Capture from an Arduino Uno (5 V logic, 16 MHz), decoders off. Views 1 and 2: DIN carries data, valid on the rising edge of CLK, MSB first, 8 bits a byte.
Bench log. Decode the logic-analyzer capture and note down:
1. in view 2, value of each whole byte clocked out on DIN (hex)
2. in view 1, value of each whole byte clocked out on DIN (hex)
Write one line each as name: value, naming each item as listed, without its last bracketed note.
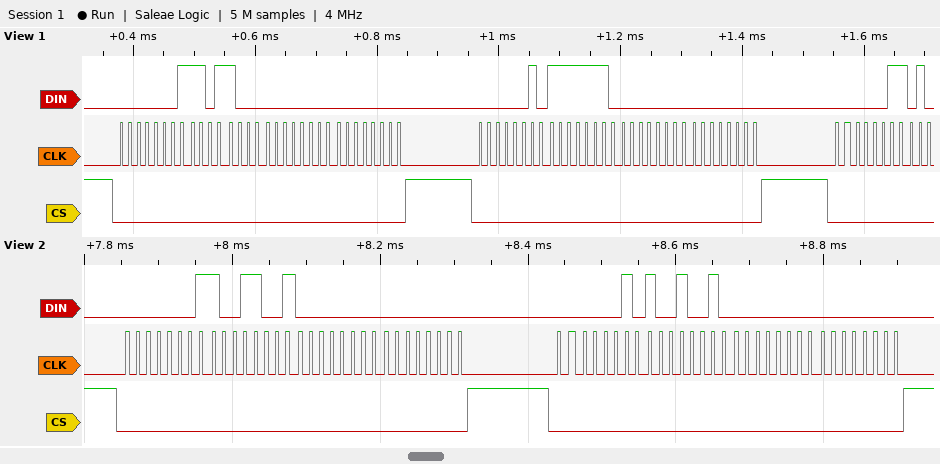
in view 2, value of each whole byte clocked out on DIN: 01 99 00 00 02 92 00 00
in view 1, value of each whole byte clocked out on DIN: 01 D8 00 00 02 FE 00 00 03
